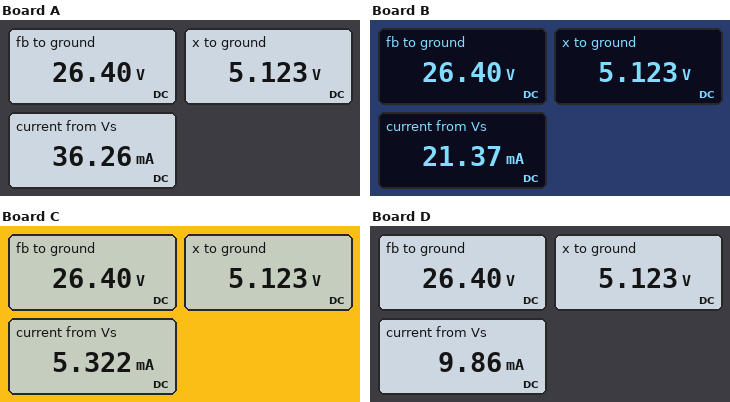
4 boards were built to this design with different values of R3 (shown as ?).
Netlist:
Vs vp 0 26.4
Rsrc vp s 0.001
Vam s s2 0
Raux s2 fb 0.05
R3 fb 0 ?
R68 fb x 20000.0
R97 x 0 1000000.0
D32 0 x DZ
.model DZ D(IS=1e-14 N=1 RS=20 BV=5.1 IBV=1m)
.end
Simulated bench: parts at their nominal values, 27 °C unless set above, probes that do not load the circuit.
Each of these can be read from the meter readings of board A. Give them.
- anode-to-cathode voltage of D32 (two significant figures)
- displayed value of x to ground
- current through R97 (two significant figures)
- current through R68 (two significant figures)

-5.1 V
5.123 V
5.1 µA
1.1 mA
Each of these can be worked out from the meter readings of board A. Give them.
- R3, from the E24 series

750 Ω
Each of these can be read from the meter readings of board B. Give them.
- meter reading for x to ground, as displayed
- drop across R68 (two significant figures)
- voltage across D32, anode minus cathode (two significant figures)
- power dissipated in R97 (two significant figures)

5.123 V
21 V
-5.1 V
26 µW
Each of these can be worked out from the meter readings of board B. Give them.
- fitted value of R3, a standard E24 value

1.3 kΩ
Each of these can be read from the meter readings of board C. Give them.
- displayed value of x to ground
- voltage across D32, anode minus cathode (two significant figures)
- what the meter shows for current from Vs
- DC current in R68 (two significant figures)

5.123 V
-5.1 V
5.322 mA
1.1 mA
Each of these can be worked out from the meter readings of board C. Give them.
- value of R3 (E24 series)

6.2 kΩ
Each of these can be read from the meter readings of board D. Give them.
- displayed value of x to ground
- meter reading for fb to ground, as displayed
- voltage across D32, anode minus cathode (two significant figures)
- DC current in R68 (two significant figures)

5.123 V
26.40 V
-5.1 V
1.1 mA
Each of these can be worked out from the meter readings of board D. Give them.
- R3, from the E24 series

3 kΩ
